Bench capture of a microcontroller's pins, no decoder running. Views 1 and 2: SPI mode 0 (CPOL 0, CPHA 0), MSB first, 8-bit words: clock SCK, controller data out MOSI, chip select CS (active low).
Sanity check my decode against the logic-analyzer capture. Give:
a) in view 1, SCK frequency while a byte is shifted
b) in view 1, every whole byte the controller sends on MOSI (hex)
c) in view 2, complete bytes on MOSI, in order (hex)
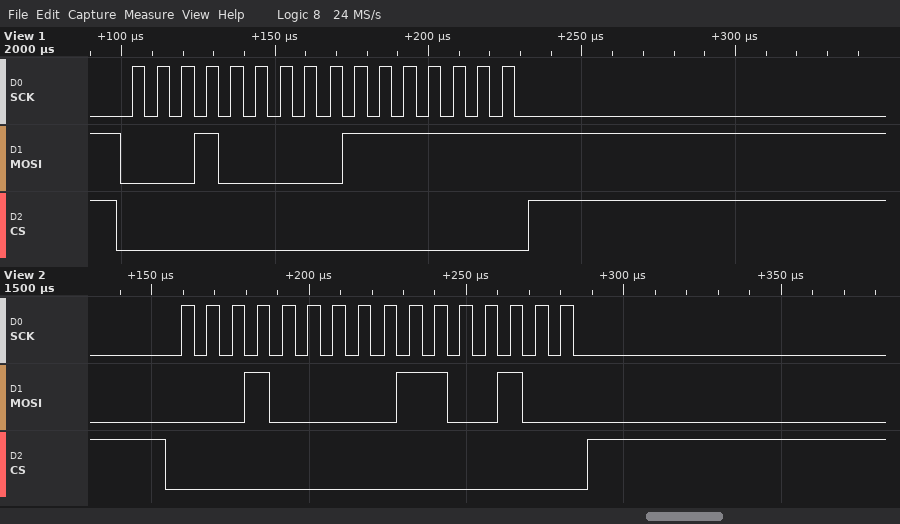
125 kHz
10 7F
10 64
